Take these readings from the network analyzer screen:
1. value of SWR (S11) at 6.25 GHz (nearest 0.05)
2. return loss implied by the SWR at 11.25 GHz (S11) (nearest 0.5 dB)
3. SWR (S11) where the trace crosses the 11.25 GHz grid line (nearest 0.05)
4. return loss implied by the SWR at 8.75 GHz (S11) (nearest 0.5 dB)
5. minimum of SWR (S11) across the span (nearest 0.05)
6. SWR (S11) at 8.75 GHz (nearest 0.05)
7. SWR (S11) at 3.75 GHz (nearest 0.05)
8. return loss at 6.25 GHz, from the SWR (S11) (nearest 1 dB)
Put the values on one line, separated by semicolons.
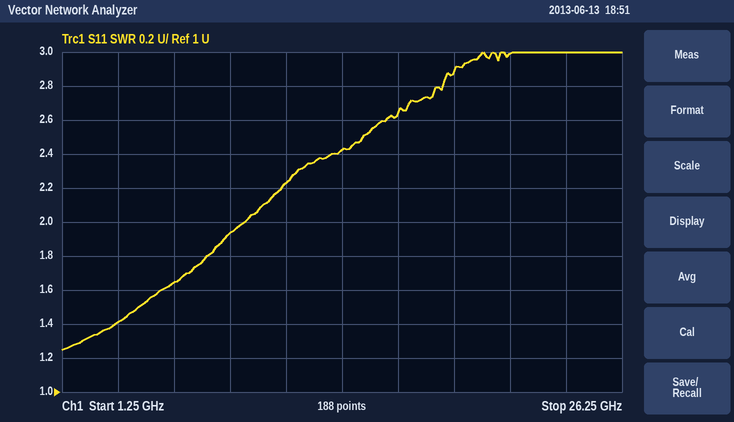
1.65; 8.5 dB; 2.25; 10.0 dB; 1.25; 1.95; 1.40; 12 dB
